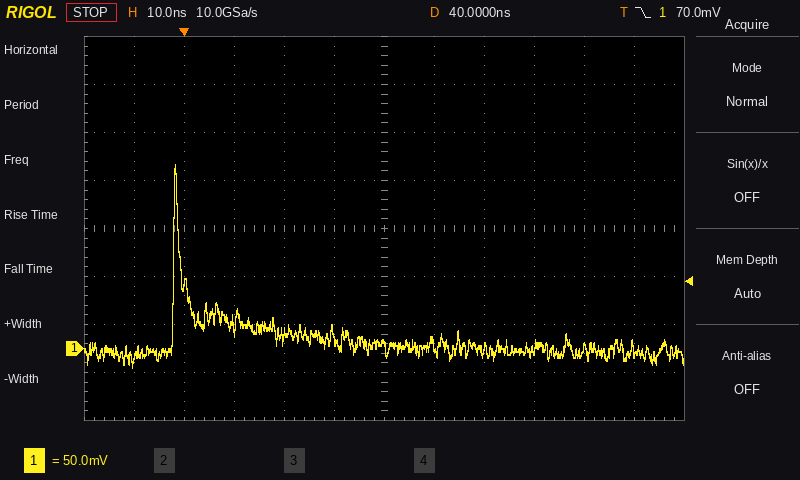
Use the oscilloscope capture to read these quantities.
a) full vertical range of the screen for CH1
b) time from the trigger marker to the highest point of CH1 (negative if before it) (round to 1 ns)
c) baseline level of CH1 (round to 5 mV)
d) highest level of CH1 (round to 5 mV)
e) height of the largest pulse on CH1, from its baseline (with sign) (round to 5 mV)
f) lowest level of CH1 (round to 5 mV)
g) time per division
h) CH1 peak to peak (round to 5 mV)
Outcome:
400 mV
-2 ns
0 mV
190 mV
+190 mV
-20 mV
10 ns
210 mV
